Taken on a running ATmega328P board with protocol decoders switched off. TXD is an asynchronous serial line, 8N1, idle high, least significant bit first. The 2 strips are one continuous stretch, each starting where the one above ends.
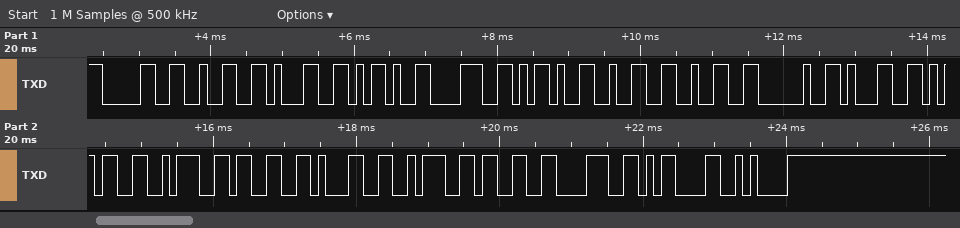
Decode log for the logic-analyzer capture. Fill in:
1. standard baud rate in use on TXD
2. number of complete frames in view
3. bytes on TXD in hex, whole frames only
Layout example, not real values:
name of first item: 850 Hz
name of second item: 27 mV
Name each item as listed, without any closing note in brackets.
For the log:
standard baud rate in use on TXD: 9600 baud
number of complete frames in view: 19
bytes on TXD in hex, whole frames only: 0x30 0x32 0x31 0x2D 0x38 0x2D 0x32 0x32 0x20 0x31 0x35 0x3A 0x33 0x31 0x3A 0x33 0x38 0x0D 0x0A
